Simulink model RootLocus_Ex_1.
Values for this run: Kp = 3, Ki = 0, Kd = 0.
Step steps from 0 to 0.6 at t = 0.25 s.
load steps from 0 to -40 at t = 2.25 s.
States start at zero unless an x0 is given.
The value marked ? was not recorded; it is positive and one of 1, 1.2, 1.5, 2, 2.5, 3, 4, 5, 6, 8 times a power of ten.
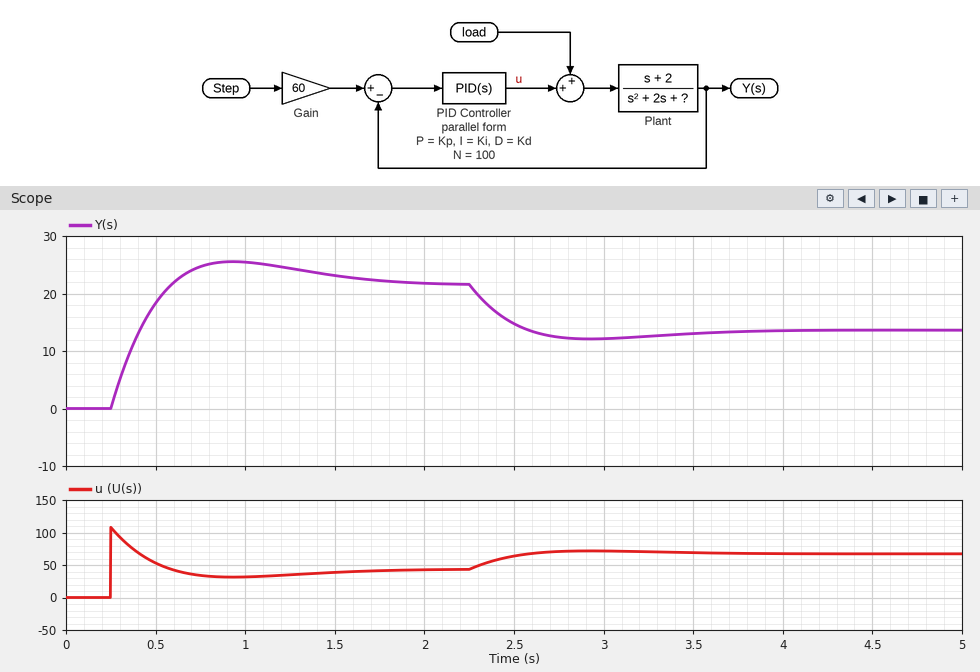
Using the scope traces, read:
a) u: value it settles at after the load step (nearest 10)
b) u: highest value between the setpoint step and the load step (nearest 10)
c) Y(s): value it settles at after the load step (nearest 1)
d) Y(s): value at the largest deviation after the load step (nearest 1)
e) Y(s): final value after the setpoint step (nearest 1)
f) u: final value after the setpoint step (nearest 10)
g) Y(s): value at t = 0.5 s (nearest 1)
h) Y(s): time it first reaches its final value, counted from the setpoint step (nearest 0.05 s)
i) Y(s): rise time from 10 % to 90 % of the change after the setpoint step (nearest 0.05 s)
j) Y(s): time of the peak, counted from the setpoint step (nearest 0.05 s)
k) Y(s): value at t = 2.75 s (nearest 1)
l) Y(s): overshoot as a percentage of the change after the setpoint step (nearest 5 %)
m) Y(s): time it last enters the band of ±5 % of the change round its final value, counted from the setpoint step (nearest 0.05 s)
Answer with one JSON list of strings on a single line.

["70", "110", "14", "12", "22", "40", "18", "0.35 s", "0.25 s", "0.70 s", "12", "20 %", "1.35 s"]
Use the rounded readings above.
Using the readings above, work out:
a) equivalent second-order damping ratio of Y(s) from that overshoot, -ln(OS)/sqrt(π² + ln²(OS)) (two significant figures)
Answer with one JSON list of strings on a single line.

["0.46"]
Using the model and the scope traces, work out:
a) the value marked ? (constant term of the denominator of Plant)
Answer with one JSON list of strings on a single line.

["4"]
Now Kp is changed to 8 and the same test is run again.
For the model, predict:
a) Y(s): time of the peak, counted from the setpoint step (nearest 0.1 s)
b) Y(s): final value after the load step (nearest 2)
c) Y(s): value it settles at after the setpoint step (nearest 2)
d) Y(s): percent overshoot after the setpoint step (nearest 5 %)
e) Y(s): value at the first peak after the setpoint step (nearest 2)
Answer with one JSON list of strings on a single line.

["0.4 s", "24", "28", "10 %", "32"]
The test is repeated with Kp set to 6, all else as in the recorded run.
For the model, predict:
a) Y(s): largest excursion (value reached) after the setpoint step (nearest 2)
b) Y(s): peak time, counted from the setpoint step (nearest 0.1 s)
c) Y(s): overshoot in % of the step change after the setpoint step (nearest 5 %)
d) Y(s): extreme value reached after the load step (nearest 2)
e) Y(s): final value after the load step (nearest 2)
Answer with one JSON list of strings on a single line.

["30", "0.5 s", "15 %", "22", "22"]
